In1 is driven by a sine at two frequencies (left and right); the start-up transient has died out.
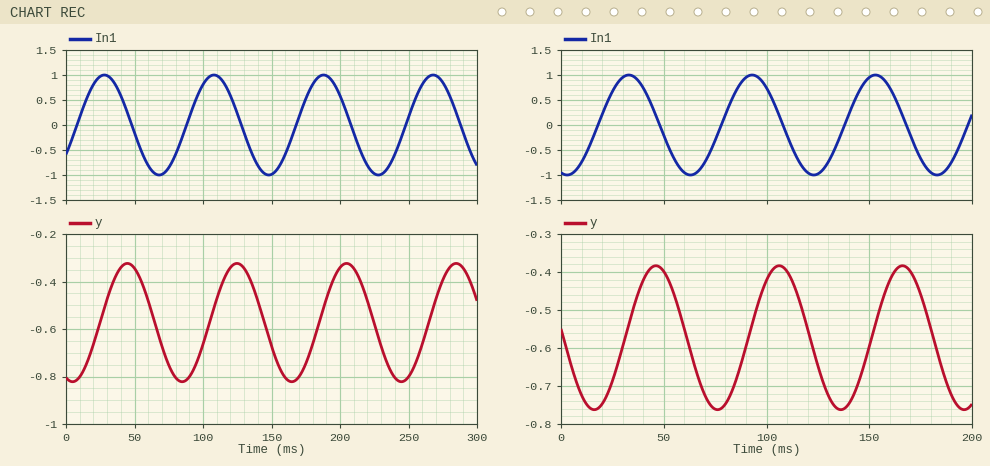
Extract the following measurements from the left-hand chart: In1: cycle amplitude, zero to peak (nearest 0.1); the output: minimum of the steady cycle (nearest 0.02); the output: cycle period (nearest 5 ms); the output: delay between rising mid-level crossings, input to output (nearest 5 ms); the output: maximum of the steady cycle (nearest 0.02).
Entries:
1.0
-0.82
80 ms
15 ms
-0.32
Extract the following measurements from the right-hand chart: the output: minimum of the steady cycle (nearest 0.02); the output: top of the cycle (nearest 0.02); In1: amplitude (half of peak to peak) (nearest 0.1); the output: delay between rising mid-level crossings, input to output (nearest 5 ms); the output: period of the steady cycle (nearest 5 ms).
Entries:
-0.76
-0.38
1.0
15 ms
60 ms
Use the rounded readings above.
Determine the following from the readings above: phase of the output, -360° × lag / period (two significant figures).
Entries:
-90°
